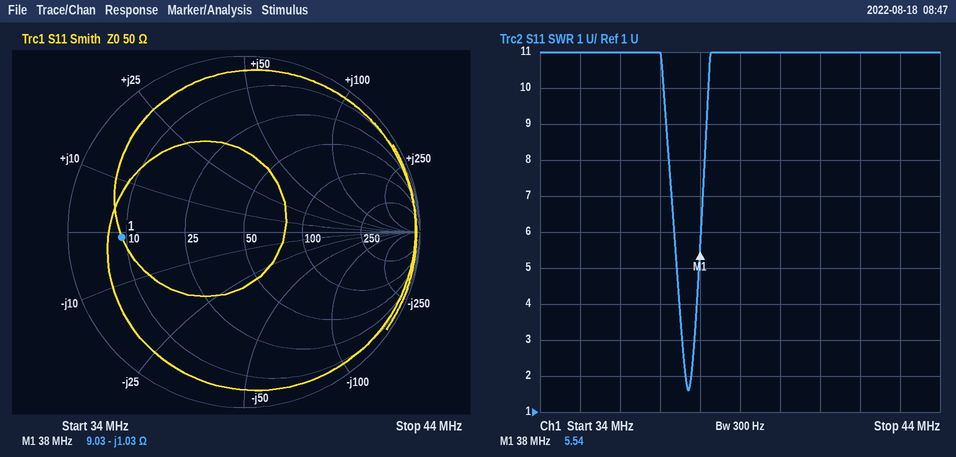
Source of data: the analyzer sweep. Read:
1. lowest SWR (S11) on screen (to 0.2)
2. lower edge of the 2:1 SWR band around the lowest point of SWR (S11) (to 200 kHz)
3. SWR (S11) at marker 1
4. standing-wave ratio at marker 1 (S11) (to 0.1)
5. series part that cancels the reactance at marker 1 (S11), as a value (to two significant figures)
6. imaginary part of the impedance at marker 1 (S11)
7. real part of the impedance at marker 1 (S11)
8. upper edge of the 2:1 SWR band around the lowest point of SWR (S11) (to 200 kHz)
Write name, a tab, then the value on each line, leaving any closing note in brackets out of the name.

lowest SWR (S11) on screen	1.6
lower edge of the 2:1 SWR band around the lowest point of SWR (S11)	37.6 MHz
SWR (S11) at marker 1	5.54
standing-wave ratio at marker 1 (S11)	5.5
series part that cancels the reactance at marker 1 (S11), as a value	4.3 nH
imaginary part of the impedance at marker 1	-1.03 Ω
real part of the impedance at marker 1	9.03 Ω
upper edge of the 2:1 SWR band around the lowest point of SWR (S11)	37.8 MHz
